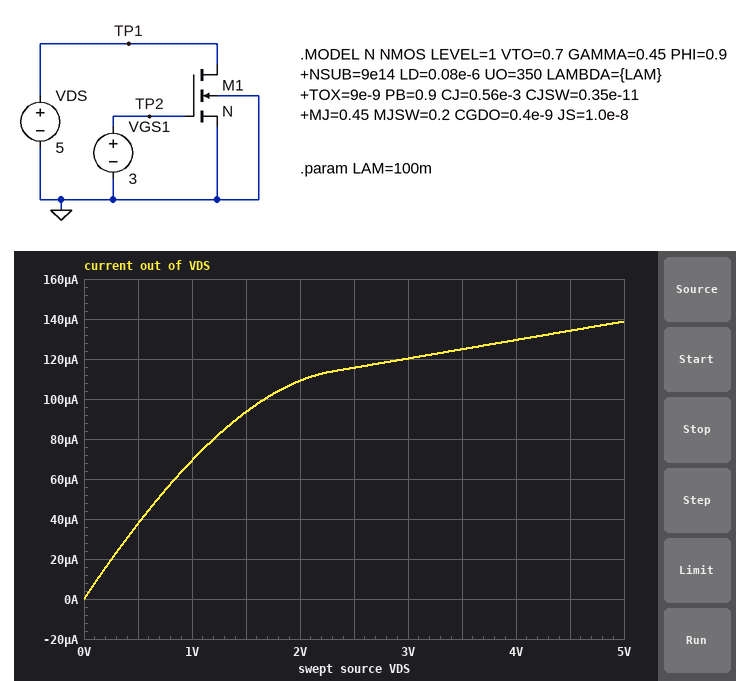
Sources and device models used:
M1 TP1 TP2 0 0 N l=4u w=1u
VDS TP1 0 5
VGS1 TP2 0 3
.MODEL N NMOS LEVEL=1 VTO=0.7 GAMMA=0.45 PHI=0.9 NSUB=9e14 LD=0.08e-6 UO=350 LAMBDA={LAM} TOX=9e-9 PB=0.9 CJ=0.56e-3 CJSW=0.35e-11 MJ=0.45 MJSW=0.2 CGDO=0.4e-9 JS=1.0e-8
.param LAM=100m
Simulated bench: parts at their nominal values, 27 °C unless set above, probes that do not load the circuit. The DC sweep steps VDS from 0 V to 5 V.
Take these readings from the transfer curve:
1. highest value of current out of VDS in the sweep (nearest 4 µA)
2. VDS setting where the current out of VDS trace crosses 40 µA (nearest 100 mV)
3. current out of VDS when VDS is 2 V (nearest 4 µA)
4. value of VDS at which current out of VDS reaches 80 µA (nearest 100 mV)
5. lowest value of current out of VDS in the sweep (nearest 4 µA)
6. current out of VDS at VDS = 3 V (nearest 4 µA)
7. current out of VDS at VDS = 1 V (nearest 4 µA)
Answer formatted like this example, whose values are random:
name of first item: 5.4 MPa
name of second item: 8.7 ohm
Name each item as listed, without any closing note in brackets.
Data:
highest value of current out of VDS in the sweep: 140 µA
VDS setting where the current out of VDS trace crosses 40 µA: 500 mV
current out of VDS when VDS is 2 V: 108 µA
value of VDS at which current out of VDS reaches 80 µA: 1.2 V
lowest value of current out of VDS in the sweep: 0 A
current out of VDS at VDS = 3 V: 120 µA
current out of VDS at VDS = 1 V: 68 µA
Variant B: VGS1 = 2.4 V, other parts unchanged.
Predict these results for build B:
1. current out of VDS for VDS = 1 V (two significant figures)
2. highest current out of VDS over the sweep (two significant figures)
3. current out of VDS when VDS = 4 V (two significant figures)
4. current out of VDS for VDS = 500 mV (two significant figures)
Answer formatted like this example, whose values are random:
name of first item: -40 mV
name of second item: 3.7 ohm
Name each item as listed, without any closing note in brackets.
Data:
current out of VDS for VDS = 1 V: 46 µA
highest current out of VDS over the sweep: 76 µA
current out of VDS when VDS = 4 V: 71 µA
current out of VDS for VDS = 500 mV: 27 µA
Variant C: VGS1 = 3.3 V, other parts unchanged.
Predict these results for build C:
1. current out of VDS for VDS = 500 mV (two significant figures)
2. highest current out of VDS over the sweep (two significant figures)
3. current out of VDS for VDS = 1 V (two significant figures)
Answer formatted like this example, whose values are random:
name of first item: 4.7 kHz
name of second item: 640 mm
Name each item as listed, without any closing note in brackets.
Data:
current out of VDS for VDS = 500 mV: 43 µA
highest current out of VDS over the sweep: 180 µA
current out of VDS for VDS = 1 V: 81 µA
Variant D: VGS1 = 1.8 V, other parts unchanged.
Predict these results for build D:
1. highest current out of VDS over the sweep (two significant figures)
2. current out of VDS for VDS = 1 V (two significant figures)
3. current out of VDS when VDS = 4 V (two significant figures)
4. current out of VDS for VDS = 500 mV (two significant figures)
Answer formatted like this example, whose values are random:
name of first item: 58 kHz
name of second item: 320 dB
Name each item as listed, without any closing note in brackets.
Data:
highest current out of VDS over the sweep: 32 µA
current out of VDS for VDS = 1 V: 23 µA
current out of VDS when VDS = 4 V: 30 µA
current out of VDS for VDS = 500 mV: 16 µA
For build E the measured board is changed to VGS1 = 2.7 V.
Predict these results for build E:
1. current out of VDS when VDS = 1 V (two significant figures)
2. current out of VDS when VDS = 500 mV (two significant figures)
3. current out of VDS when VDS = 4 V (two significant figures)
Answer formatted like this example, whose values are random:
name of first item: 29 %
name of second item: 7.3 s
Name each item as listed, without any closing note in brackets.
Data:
current out of VDS when VDS = 1 V: 58 µA
current out of VDS when VDS = 500 mV: 32 µA
current out of VDS when VDS = 4 V: 98 µA
